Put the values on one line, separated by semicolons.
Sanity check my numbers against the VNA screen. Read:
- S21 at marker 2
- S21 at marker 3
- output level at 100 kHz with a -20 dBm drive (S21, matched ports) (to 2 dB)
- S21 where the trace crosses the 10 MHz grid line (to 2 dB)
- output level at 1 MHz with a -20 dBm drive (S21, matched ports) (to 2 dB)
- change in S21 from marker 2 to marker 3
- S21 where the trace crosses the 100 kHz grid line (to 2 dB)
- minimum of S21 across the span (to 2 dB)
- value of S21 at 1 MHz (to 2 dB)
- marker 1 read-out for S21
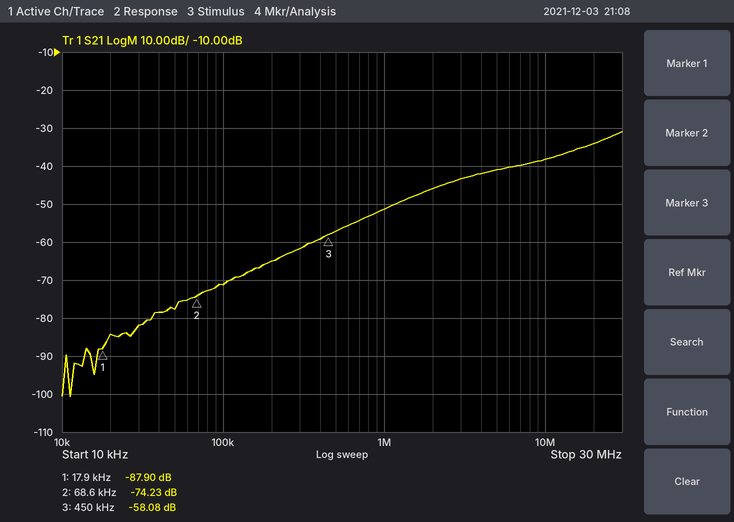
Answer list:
-74.23 dB; -58.08 dB; -92 dBm; -38 dB; -72 dBm; 16.15 dB; -72 dB; -100 dB; -52 dB; -87.90 dB
